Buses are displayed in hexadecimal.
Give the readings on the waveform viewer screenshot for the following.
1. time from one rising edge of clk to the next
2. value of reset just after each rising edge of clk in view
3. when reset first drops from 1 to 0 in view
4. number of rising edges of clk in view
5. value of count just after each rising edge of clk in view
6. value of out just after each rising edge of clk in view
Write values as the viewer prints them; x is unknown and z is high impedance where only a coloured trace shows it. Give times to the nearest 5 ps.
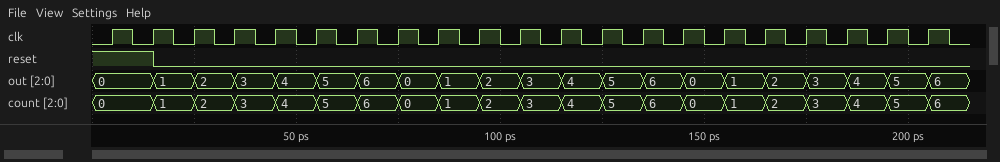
10 ps
1 0 0 0 0 0 0 0 0 0 0 0 0 0 0 0 0 0 0 0 0
15 ps
21
0, 1, 2, 3, 4, 5, 6, 0, 1, 2, 3, 4, 5, 6, 0, 1, 2, 3, 4, 5, 6
0, 1, 2, 3, 4, 5, 6, 0, 1, 2, 3, 4, 5, 6, 0, 1, 2, 3, 4, 5, 6
